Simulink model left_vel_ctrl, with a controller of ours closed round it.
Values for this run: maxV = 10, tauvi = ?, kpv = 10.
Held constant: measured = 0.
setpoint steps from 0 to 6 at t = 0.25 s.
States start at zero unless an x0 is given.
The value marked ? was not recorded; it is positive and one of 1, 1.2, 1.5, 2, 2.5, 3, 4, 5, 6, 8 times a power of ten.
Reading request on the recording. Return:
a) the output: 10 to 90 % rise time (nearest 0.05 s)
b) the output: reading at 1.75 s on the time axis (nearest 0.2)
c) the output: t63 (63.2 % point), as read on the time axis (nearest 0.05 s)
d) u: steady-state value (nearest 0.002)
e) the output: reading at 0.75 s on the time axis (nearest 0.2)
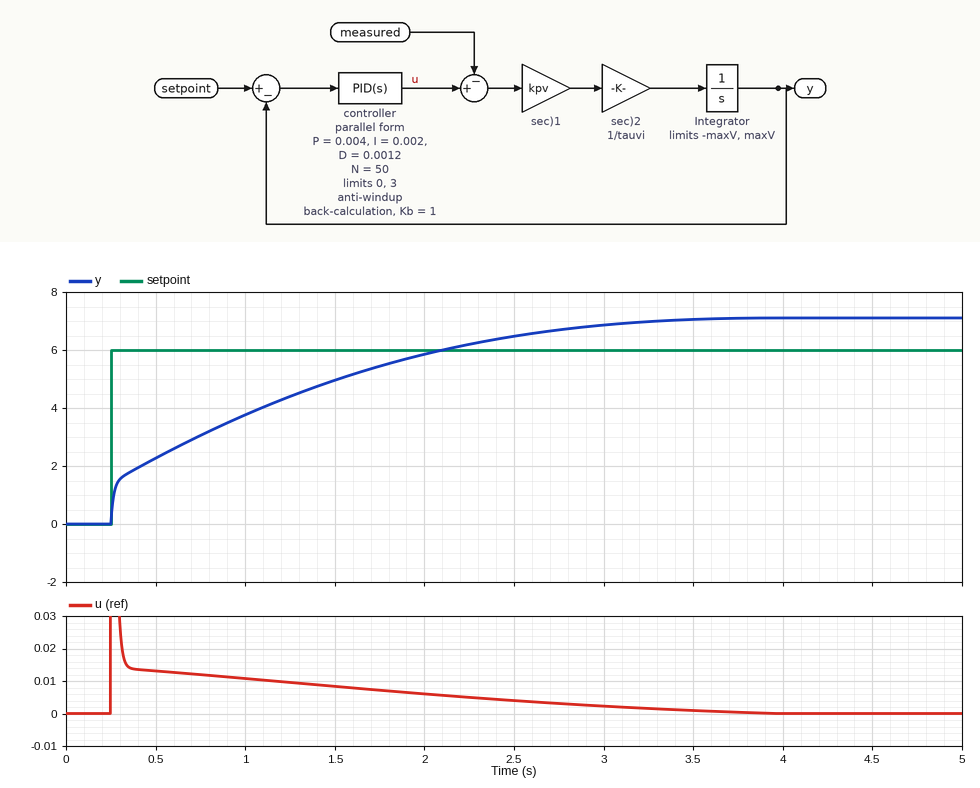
2.15 s
5.4
1.30 s
0.000
3.0
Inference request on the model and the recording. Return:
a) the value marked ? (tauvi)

0.04
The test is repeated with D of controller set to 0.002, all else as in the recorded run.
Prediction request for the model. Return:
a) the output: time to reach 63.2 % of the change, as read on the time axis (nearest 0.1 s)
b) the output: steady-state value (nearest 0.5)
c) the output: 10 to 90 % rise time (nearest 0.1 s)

1.3 s
7.0
2.3 s
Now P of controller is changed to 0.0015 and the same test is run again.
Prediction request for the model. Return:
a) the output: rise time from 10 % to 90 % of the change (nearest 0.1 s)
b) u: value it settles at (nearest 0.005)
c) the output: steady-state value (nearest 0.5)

3.1 s
0.000
8.5
